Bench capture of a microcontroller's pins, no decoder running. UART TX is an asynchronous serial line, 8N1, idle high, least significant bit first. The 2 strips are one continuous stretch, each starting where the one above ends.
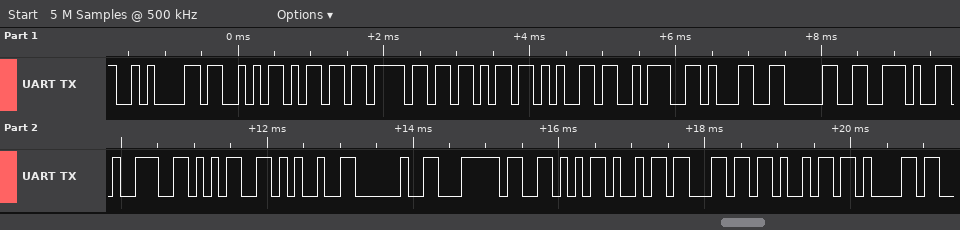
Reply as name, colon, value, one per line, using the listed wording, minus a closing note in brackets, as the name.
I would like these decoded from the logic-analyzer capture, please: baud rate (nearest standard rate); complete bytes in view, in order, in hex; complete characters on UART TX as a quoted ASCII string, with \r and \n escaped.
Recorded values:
baud rate: 9600 baud
complete bytes in view, in order, in hex: 0A 53 6D 6F 6B 65 3A 31 30 2E 39 35 25 20 7C 56 69 6C 69 61
complete characters on UART TX as a quoted ASCII string, with \r and \n escaped: "\nSmoke:10.95% |Vilia"
